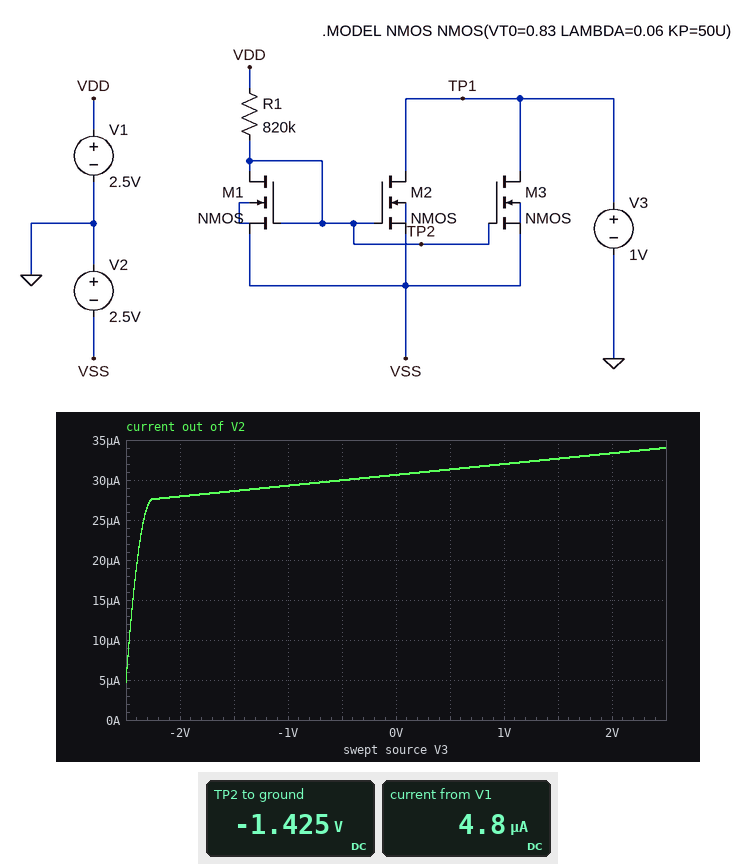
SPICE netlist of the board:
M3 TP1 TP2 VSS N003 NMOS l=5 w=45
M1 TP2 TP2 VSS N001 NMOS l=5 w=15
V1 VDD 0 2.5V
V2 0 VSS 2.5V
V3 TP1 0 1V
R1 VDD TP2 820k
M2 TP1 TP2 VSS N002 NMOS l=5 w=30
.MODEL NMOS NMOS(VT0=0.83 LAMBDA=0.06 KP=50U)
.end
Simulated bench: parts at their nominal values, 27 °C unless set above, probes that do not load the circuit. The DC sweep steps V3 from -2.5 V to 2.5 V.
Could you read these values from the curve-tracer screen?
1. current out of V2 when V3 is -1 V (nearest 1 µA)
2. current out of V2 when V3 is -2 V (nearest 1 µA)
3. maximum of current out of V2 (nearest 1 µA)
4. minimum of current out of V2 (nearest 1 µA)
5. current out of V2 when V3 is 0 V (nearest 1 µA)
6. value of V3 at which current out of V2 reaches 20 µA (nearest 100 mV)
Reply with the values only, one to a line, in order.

29 µA
28 µA
34 µA
5 µA
31 µA
-2.4 V
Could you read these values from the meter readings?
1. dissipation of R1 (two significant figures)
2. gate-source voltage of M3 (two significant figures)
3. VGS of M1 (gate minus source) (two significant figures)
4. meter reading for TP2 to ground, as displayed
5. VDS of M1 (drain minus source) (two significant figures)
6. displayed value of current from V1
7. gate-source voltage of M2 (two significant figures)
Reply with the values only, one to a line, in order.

19 µW
1.1 V
1.1 V
-1.425 V
1.1 V
4.8 µA
1.1 V
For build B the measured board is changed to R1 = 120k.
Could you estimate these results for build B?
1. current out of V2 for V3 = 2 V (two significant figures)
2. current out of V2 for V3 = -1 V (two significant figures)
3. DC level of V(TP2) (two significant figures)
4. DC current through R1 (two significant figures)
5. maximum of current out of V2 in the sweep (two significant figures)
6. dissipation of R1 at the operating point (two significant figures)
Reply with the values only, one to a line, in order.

200 µA
180 µA
-1.1 V
30 µA
210 µA
110 µW
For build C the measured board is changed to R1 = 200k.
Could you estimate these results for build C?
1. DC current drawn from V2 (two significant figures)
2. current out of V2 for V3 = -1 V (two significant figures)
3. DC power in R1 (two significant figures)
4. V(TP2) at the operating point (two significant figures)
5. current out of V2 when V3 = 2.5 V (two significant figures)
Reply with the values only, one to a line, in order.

120 µA
110 µA
68 µW
-1.2 V
130 µA
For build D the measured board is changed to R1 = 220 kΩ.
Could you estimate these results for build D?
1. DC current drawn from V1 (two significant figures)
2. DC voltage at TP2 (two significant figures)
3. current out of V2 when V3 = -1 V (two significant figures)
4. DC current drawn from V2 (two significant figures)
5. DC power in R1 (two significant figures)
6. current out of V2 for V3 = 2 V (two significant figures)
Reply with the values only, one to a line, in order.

17 µA
-1.2 V
100 µA
110 µA
63 µW
120 µA
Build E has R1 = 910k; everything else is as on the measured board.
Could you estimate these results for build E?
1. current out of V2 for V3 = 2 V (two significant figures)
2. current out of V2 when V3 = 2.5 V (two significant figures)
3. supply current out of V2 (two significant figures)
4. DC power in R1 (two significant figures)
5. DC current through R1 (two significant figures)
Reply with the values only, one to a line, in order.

30 µA
31 µA
29 µA
17 µW
4.3 µA
